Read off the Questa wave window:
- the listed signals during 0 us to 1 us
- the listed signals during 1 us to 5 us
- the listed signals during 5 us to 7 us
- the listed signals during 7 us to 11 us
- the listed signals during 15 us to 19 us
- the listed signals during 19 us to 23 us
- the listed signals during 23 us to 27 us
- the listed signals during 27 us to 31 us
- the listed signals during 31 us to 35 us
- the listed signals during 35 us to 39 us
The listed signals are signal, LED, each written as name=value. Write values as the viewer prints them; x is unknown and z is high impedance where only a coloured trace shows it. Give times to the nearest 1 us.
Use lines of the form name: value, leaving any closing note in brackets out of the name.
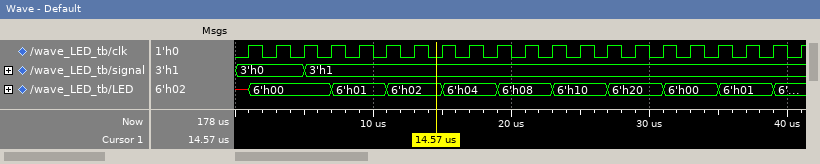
the listed signals during 0 us to 1 us: signal=3'h0, LED=x
the listed signals during 1 us to 5 us: signal=3'h0, LED=6'h00
the listed signals during 5 us to 7 us: signal=3'h1, LED=6'h00
the listed signals during 7 us to 11 us: signal=3'h1, LED=6'h01
the listed signals during 15 us to 19 us: signal=3'h1, LED=6'h04
the listed signals during 19 us to 23 us: signal=3'h1, LED=6'h08
the listed signals during 23 us to 27 us: signal=3'h1, LED=6'h10
the listed signals during 27 us to 31 us: signal=3'h1, LED=6'h20
the listed signals during 31 us to 35 us: signal=3'h1, LED=6'h00
the listed signals during 35 us to 39 us: signal=3'h1, LED=6'h01
